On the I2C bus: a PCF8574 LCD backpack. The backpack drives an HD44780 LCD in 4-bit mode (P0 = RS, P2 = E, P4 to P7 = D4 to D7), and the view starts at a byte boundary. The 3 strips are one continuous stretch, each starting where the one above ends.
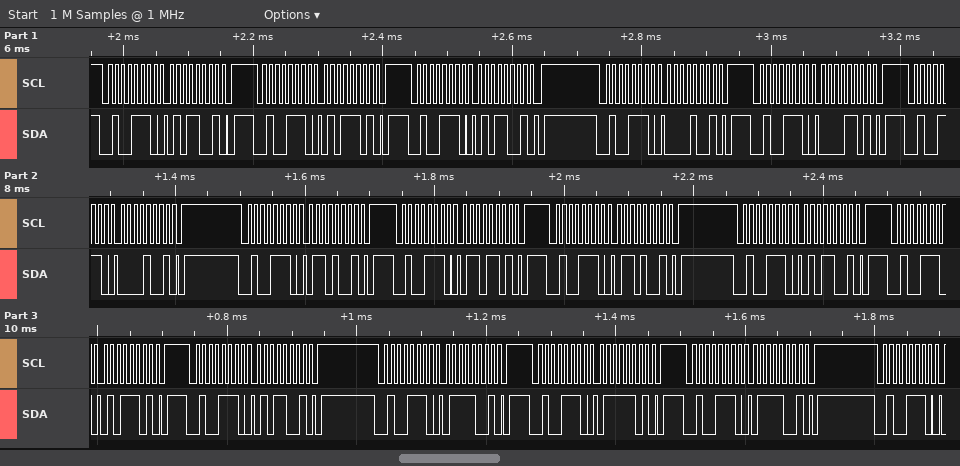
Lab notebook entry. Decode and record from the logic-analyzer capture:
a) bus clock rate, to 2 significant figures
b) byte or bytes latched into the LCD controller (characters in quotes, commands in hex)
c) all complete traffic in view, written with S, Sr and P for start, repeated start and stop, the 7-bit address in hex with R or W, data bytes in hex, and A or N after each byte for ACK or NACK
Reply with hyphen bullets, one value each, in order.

- 100 kHz
- 'P' 'e'
- S 27W A 59 A P S 27W A 5D A P S 27W A 59 A P S 27W A 09 A P S 27W A 0D A P S 27W A 09 A P S 27W A 69 A P S 27W A 6D A P S 27W A 69 A P S 27W A 59 A P S 27W A 5D A P S 27W A 59 A P S 27W A 79 A P S 27W A 7D A P S 27W A 79 A P S 27W A
